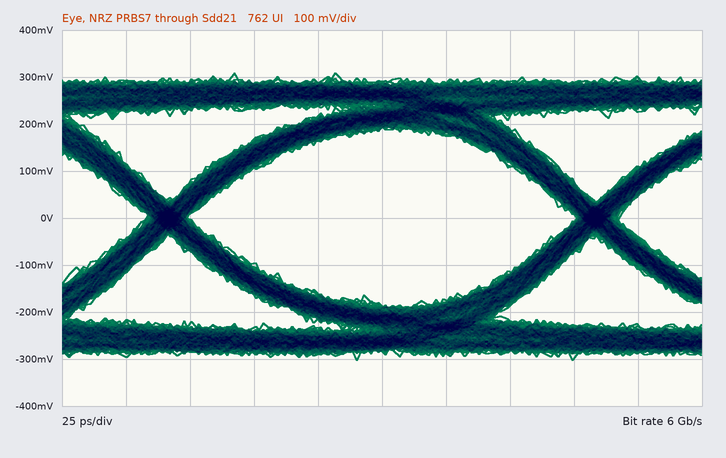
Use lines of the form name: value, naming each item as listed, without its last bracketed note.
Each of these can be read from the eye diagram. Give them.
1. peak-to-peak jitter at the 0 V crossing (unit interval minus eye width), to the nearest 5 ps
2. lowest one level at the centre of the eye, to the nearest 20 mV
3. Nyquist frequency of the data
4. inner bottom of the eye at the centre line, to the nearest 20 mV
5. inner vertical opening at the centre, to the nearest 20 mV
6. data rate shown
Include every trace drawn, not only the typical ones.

peak-to-peak jitter at the 0 V crossing (unit interval minus eye width), to the nearest 5 ps: 15 ps
lowest one level at the centre of the eye, to the nearest 20 mV: 200 mV
Nyquist frequency of the data: 3 GHz
inner bottom of the eye at the centre line, to the nearest 20 mV: -180 mV
inner vertical opening at the centre, to the nearest 20 mV: 380 mV
data rate shown: 6 Gb/s
